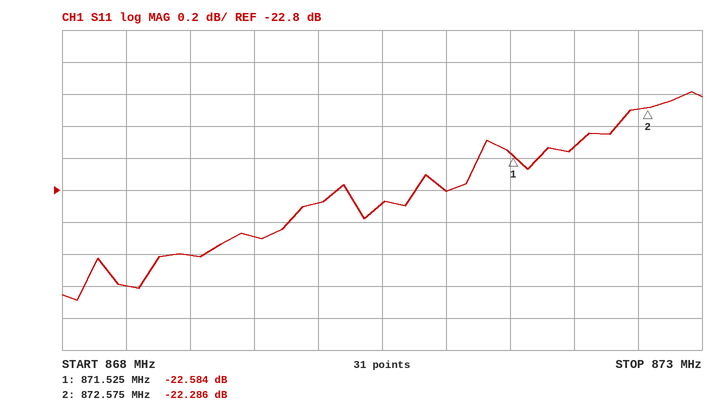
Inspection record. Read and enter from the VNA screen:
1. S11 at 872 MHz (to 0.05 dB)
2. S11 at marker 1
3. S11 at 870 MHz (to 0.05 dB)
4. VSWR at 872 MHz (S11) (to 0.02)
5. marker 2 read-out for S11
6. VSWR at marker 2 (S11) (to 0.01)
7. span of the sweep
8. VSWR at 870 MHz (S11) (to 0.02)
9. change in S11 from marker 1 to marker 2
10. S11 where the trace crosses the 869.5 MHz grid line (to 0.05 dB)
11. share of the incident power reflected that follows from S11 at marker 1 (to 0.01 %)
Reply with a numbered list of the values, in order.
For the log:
1. -22.55 dB
2. -22.584 dB
3. -22.90 dB
4. 1.16
5. -22.286 dB
6. 1.17
7. 5 MHz
8. 1.16
9. 0.298 dB
10. -23.10 dB
11. 0.55 %
